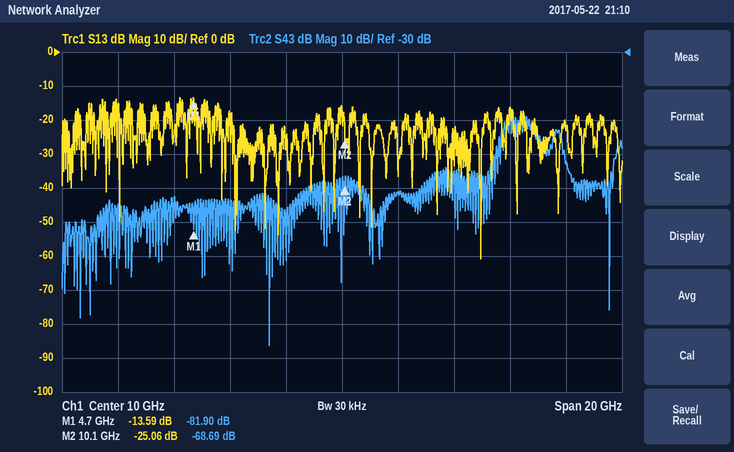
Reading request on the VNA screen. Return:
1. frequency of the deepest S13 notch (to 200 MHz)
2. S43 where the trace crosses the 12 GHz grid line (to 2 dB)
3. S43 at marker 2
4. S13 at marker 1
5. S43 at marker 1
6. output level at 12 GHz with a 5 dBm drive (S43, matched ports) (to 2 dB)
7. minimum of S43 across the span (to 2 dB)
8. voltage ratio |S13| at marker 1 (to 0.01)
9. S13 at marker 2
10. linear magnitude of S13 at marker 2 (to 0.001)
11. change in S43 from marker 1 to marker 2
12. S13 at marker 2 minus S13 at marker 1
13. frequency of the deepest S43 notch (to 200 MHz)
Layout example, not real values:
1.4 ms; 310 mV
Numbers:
15.0 GHz; -72 dB; -68.69 dB; -13.59 dB; -81.90 dB; -66 dBm; -116 dB; 0.21; -25.06 dB; 0.056; 13.21 dB; -11.47 dB; 7.4 GHz
